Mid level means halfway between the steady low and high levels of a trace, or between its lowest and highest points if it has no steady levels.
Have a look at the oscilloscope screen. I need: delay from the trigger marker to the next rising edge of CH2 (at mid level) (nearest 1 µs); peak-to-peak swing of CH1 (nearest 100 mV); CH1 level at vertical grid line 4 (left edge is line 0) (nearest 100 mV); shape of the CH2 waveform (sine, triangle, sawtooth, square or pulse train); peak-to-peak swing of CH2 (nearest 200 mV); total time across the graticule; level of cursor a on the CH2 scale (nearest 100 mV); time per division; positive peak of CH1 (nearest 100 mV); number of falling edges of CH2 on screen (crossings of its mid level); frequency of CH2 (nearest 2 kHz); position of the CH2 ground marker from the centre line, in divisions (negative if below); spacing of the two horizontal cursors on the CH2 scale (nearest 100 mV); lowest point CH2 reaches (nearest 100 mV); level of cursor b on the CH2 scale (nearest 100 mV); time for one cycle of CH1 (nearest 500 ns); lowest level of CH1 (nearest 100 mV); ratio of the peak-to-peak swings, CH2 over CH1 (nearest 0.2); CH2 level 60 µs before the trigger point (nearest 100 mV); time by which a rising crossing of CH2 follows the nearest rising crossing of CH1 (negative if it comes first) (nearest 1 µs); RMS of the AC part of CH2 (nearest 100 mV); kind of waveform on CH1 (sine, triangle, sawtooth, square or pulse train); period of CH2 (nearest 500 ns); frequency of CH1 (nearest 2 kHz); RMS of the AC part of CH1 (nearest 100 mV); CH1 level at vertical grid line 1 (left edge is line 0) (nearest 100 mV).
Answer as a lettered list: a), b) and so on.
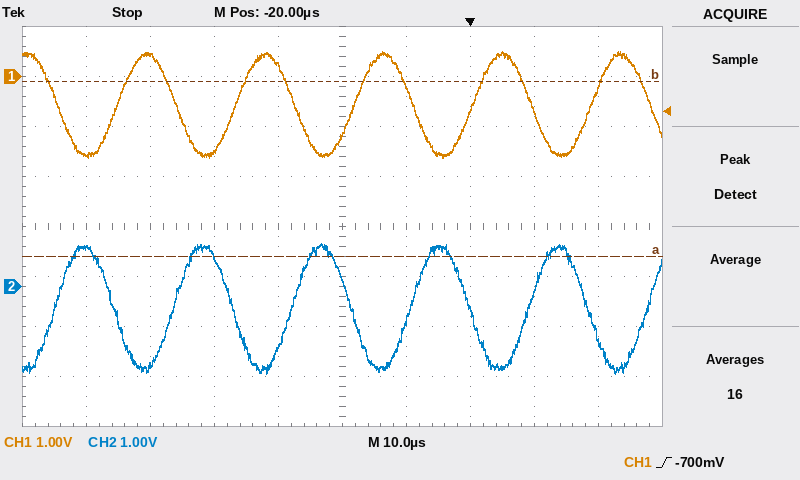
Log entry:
a) 9 µs
b) 2.1 V
c) 200 mV
d) sine
e) 2.6 V
f) 100 µs
g) 600 mV
h) 10 µs
i) 500 mV
j) 5
k) 54 kHz
l) -1.2 div
m) 3.5 V
n) -1.7 V
o) 4.1 V
p) 18.5 µs
q) -1.6 V
r) 1.2
s) 800 mV
t) +9 µs
u) 900 mV
v) sine
w) 18.5 µs
x) 54 kHz
y) 700 mV
z) -1.6 V
